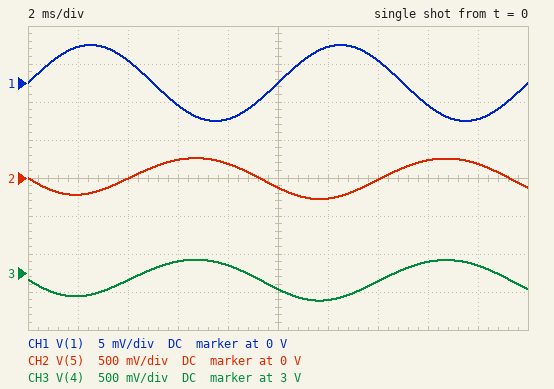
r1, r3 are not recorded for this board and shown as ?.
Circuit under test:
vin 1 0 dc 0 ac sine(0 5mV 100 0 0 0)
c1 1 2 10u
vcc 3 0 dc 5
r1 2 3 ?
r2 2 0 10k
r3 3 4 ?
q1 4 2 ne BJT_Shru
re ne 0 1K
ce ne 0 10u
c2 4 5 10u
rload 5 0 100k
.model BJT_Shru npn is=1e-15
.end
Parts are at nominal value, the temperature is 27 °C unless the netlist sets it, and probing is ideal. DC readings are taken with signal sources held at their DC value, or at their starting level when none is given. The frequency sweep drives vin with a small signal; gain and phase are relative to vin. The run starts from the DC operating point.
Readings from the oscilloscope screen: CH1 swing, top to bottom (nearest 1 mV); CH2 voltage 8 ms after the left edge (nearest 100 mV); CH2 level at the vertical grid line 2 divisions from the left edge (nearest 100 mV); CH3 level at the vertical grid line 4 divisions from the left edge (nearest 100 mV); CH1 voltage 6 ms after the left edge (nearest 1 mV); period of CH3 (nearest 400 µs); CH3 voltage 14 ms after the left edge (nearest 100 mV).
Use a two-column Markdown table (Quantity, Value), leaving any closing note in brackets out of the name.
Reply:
| Quantity | Value |
|---|---|
| CH1 swing, top to bottom | 10 mV |
| CH2 voltage 8 ms after the left edge | 200 mV |
| CH2 level at the vertical grid line 2 divisions from the left edge | 0 V |
| CH3 level at the vertical grid line 4 divisions from the left edge | 3.1 V |
| CH1 voltage 6 ms after the left edge | -3 mV |
| period of CH3 | 10.0 ms |
| CH3 voltage 14 ms after the left edge | 2.9 V |
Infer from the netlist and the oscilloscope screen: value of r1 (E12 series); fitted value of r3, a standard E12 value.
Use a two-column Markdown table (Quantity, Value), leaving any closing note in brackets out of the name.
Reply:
| Quantity | Value |
|---|---|
| value of r1 | 56 kΩ |
| fitted value of r3, a standard E12 value | 22 kΩ |
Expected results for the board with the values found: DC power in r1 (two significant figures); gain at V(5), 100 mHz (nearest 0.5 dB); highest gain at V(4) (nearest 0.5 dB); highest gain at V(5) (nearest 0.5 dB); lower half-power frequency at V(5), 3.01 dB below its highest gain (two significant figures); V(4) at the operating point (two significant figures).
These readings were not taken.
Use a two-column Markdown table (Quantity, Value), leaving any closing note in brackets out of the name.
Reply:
| Quantity | Value |
|---|---|
| DC power in r1 | 320 µW |
| gain at V(5), 100 mHz | -7.5 dB |
| highest gain at V(4) | 36.5 dB |
| highest gain at V(5) | 36.5 dB |
| lower half-power frequency at V(5), 3.01 dB below its highest gain | 72 Hz |
| V(4) at the operating point | 2.9 V |
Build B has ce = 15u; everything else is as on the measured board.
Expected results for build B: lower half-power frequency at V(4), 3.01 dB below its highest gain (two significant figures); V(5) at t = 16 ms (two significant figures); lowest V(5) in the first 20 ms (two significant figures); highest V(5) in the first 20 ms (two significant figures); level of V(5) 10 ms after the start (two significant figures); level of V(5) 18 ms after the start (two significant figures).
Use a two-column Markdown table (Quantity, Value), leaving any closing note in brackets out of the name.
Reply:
| Quantity | Value |
|---|---|
| lower half-power frequency at V(4), 3.01 dB below its highest gain | 48 Hz |
| V(5) at t = 16 ms | 240 mV |
| lowest V(5) in the first 20 ms | -310 mV |
| highest V(5) in the first 20 ms | 290 mV |
| level of V(5) 10 ms after the start | -100 mV |
| level of V(5) 18 ms after the start | 230 mV |
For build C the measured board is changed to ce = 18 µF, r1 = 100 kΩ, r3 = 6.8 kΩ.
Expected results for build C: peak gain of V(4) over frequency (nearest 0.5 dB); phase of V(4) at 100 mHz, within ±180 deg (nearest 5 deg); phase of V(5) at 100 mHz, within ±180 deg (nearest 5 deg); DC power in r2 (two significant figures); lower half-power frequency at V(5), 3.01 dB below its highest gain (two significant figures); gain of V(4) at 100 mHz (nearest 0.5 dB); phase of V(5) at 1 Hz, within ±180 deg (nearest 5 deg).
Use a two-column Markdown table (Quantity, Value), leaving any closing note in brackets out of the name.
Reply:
| Quantity | Value |
|---|---|
| peak gain of V(4) over frequency | -39.5 dB |
| phase of V(4) at 100 mHz, within ±180 deg | -95 deg |
| phase of V(5) at 100 mHz, within ±180 deg | -35 deg |
| DC power in r2 | 21 µW |
| lower half-power frequency at V(5), 3.01 dB below its highest gain | 1.8 Hz |
| gain of V(4) at 100 mHz | -64.0 dB |
| phase of V(5) at 1 Hz, within ±180 deg | -110 deg |
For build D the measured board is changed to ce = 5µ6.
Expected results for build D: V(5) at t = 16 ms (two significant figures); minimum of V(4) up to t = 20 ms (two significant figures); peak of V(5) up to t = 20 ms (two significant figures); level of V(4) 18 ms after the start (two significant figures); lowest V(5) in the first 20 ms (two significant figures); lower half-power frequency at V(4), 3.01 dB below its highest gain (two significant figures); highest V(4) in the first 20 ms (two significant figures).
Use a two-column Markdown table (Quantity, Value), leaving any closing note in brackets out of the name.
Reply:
| Quantity | Value |
|---|---|
| V(5) at t = 16 ms | 190 mV |
| minimum of V(4) up to t = 20 ms | 2.7 V |
| peak of V(5) up to t = 20 ms | 200 mV |
| level of V(4) 18 ms after the start | 3.0 V |
| lowest V(5) in the first 20 ms | -210 mV |
| lower half-power frequency at V(4), 3.01 dB below its highest gain | 130 Hz |
| highest V(4) in the first 20 ms | 3.1 V |
